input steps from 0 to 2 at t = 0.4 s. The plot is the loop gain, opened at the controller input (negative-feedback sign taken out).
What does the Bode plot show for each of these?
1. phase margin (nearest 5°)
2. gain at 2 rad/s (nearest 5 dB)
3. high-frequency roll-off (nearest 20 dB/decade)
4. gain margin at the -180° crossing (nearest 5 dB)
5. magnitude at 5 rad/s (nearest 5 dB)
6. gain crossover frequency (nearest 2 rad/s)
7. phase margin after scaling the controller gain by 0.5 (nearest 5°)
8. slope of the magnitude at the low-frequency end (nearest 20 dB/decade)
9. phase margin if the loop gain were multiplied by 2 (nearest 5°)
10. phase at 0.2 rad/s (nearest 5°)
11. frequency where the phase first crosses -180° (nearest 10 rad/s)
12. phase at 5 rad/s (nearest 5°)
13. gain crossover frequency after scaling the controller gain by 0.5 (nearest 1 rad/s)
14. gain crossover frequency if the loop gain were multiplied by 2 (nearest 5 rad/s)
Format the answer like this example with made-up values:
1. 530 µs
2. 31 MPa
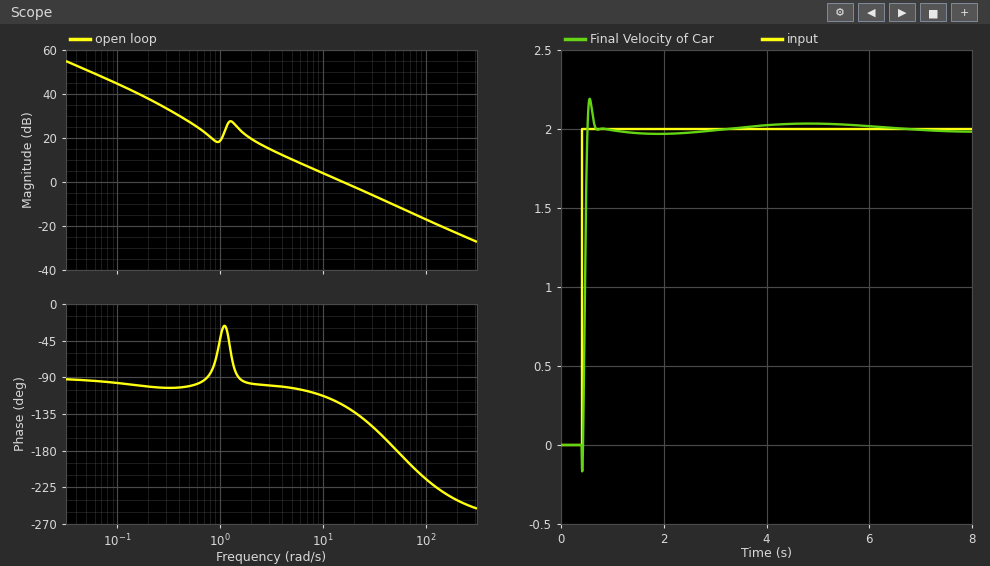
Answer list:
1. 55°
2. 20 dB
3. -20 dB/decade
4. 10 dB
5. 10 dB
6. 16 rad/s
7. 70°
8. -20 dB/decade
9. 30°
10. -100°
11. 50 rad/s
12. -105°
13. 8 rad/s
14. 30 rad/s
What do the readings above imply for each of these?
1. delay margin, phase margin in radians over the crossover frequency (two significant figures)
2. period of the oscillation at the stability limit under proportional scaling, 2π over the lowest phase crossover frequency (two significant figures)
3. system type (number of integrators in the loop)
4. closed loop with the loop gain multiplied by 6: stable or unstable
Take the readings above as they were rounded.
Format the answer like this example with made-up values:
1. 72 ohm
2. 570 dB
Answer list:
1. 0.060 s
2. 0.13 s
3. 1
4. unstable
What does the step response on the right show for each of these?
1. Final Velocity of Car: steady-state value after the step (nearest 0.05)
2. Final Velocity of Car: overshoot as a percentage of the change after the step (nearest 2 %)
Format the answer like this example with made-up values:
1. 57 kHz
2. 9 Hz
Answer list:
1. 2.00
2. 10 %
